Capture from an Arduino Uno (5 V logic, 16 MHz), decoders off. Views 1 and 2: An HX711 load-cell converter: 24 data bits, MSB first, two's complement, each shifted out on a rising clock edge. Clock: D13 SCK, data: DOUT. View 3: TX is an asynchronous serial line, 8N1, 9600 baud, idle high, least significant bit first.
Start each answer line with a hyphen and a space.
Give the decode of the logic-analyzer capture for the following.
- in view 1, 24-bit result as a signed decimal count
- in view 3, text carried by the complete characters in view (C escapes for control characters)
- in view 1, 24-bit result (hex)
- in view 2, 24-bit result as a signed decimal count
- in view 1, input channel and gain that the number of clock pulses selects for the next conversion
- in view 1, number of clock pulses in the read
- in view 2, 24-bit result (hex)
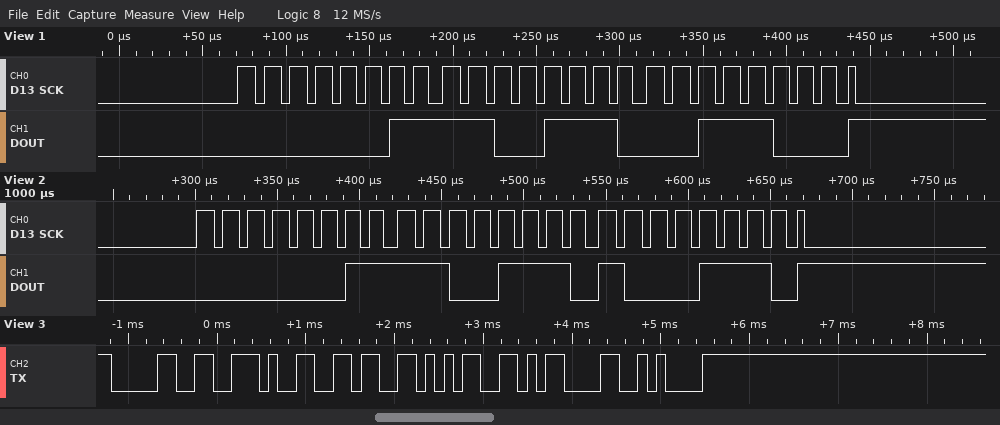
- 249400
- "0.65\r\n"
- 0x03CE38
- 249486
- channel A, gain 128
- 25
- 0x03CE8E
